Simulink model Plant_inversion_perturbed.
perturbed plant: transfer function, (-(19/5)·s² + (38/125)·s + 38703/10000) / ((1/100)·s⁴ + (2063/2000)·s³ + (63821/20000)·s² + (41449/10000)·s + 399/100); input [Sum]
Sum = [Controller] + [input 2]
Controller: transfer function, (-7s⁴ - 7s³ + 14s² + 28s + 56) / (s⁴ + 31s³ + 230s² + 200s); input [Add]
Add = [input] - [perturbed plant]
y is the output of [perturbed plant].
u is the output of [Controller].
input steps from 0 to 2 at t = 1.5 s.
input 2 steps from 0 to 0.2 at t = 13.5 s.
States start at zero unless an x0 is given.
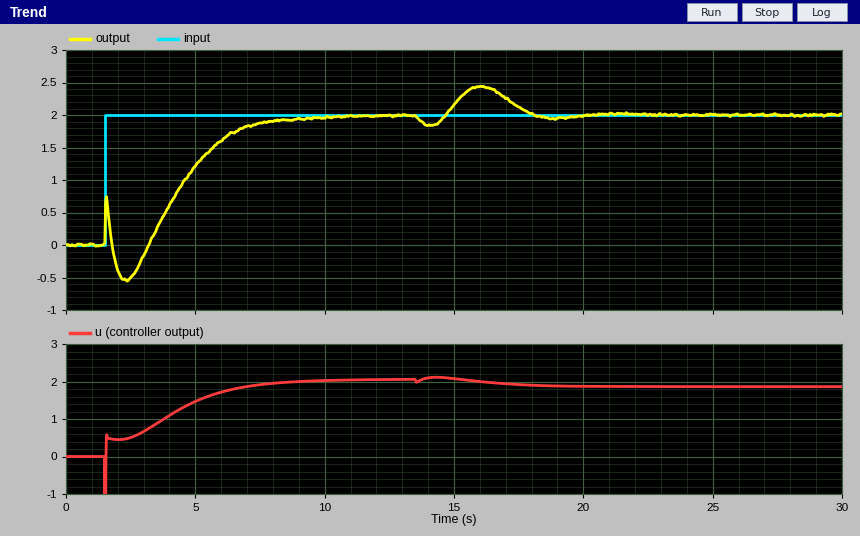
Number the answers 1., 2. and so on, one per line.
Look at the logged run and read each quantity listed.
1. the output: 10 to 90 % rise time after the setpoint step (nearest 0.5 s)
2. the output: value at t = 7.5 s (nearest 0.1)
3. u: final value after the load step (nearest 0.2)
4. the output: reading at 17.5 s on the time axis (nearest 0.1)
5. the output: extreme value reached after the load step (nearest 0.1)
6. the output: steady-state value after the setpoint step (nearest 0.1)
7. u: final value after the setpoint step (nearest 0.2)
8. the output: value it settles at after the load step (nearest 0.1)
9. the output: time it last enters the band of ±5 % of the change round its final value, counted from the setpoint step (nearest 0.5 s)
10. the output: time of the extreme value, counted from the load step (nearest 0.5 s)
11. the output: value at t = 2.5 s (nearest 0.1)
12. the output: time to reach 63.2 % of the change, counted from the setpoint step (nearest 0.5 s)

1. 5.5 s
2. 1.9
3. 1.8
4. 2.1
5. 2.4
6. 2.0
7. 2.0
8. 2.0
9. 6.5 s
10. 2.5 s
11. -0.5
12. 3.5 s
